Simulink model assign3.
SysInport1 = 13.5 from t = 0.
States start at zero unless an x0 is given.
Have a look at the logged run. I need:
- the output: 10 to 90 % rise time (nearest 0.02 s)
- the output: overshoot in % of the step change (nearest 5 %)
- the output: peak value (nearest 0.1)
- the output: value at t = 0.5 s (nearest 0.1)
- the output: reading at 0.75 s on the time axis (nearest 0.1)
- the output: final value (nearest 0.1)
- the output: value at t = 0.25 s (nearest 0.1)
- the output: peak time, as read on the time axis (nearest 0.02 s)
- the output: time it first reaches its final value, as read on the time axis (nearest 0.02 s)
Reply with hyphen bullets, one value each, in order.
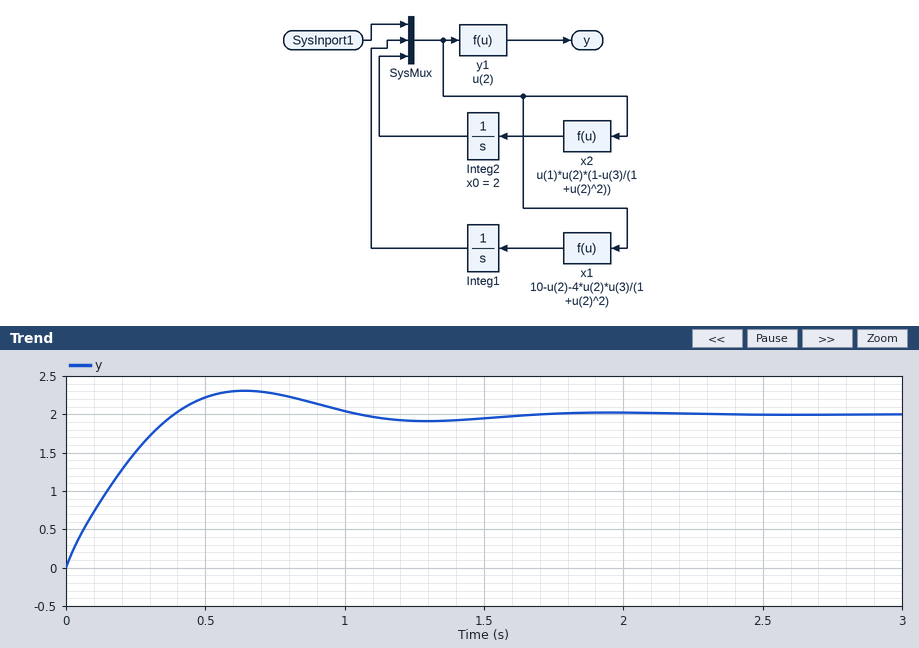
- 0.30 s
- 15 %
- 2.3
- 2.2
- 2.3
- 2.0
- 1.5
- 0.64 s
- 0.38 s
